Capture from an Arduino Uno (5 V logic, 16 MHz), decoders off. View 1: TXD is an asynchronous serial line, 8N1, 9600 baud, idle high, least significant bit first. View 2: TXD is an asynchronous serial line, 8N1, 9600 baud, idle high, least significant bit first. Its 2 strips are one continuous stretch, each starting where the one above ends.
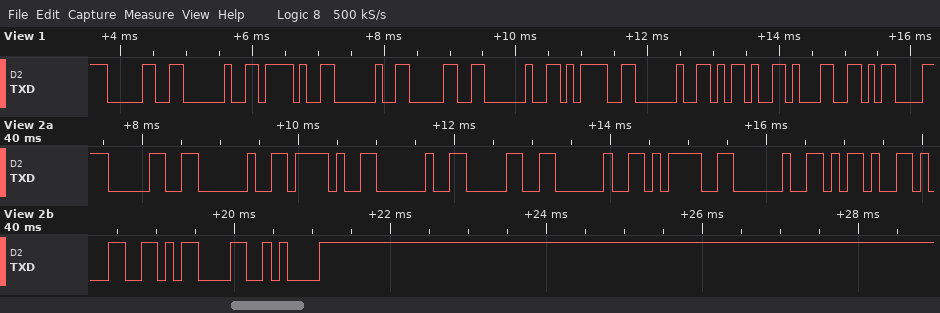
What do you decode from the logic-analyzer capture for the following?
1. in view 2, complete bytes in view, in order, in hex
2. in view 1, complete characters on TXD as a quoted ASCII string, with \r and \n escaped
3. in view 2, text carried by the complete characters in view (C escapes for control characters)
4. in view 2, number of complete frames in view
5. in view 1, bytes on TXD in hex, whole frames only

30 20 2F 20 30 20 3D 20 2D 31 0D 0A
"0 / 0 = -1\r"
"0 / 0 = -1\r\n"
12
30 20 2F 20 30 20 3D 20 2D 31 0D
